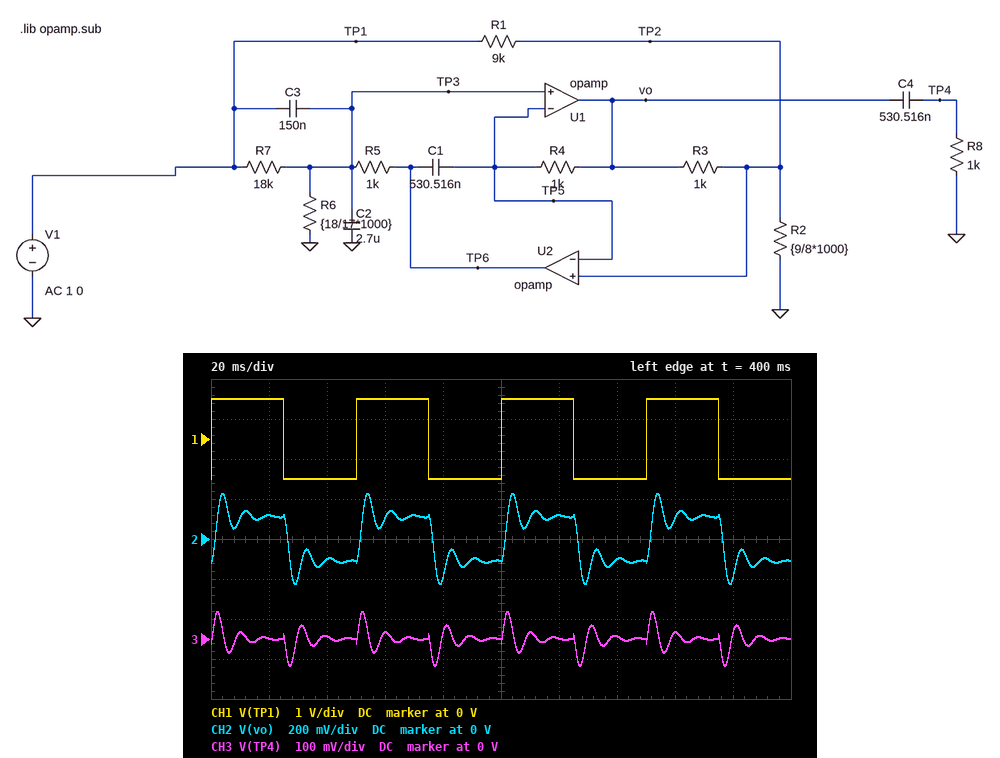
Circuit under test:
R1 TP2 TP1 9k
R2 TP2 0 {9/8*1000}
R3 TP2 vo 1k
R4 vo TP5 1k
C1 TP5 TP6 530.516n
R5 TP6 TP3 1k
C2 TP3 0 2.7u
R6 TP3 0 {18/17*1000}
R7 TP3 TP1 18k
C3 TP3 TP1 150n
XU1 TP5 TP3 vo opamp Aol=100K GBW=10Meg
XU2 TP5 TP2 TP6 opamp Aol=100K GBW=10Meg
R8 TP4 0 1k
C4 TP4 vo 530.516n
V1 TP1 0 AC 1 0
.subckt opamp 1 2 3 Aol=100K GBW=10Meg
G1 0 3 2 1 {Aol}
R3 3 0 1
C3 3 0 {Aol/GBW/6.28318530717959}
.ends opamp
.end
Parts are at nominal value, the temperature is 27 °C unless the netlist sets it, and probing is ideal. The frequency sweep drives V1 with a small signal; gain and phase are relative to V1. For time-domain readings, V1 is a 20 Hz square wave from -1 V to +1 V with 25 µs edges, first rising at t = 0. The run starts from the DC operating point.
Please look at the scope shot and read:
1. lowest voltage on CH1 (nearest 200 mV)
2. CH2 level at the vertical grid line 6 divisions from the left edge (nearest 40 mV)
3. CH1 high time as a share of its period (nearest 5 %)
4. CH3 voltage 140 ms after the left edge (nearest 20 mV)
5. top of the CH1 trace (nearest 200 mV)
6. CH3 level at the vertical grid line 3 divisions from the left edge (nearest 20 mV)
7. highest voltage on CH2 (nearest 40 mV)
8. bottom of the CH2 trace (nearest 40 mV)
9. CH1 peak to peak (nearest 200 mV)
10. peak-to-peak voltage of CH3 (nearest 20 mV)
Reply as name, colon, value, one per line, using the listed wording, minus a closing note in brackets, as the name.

lowest voltage on CH1: -1.0 V
CH2 level at the vertical grid line 6 divisions from the left edge: 120 mV
CH1 high time as a share of its period: 50 %
CH3 voltage 140 ms after the left edge: 0 V
top of the CH1 trace: 1.0 V
CH3 level at the vertical grid line 3 divisions from the left edge: 20 mV
highest voltage on CH2: 240 mV
bottom of the CH2 trace: -240 mV
CH1 peak to peak: 2.0 V
peak-to-peak voltage of CH3: 140 mV
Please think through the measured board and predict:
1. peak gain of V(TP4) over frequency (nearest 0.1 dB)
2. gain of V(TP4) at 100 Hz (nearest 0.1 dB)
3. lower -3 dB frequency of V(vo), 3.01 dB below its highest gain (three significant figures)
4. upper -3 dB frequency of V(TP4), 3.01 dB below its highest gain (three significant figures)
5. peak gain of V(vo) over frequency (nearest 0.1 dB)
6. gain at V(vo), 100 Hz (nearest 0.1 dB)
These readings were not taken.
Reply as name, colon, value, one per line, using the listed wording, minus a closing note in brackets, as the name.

peak gain of V(TP4) over frequency: -19.4 dB
gain of V(TP4) at 100 Hz: -23.2 dB
lower -3 dB frequency of V(vo), 3.01 dB below its highest gain: 91.8 Hz
upper -3 dB frequency of V(TP4), 3.01 dB below its highest gain: 159 Hz
peak gain of V(vo) over frequency: -11.2 dB
gain at V(vo), 100 Hz: -13.2 dB
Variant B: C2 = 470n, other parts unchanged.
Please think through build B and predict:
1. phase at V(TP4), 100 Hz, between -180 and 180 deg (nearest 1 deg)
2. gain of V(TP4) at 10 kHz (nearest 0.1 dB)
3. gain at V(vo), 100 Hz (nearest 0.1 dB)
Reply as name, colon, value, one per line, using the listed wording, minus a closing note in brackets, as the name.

phase at V(TP4), 100 Hz, between -180 and 180 deg: 51 deg
gain of V(TP4) at 10 kHz: -8.6 dB
gain at V(vo), 100 Hz: -23.4 dB
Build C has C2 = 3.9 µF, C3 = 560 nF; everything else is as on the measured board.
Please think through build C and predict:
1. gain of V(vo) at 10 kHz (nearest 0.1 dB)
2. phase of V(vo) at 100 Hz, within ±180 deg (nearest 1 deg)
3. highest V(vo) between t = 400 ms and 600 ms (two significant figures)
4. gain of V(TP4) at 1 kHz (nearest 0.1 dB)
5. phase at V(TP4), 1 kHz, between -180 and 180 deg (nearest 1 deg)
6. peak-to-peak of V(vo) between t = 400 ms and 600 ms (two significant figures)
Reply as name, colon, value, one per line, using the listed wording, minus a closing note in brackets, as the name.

gain of V(vo) at 10 kHz: -17.1 dB
phase of V(vo) at 100 Hz, within ±180 deg: 101 deg
highest V(vo) between t = 400 ms and 600 ms: 170 mV
gain of V(TP4) at 1 kHz: -17.4 dB
phase at V(TP4), 1 kHz, between -180 and 180 deg: 19 deg
peak-to-peak of V(vo) between t = 400 ms and 600 ms: 340 mV
